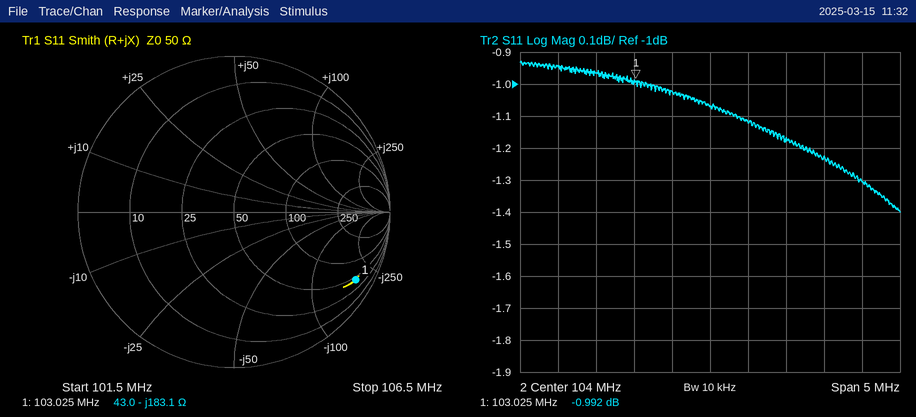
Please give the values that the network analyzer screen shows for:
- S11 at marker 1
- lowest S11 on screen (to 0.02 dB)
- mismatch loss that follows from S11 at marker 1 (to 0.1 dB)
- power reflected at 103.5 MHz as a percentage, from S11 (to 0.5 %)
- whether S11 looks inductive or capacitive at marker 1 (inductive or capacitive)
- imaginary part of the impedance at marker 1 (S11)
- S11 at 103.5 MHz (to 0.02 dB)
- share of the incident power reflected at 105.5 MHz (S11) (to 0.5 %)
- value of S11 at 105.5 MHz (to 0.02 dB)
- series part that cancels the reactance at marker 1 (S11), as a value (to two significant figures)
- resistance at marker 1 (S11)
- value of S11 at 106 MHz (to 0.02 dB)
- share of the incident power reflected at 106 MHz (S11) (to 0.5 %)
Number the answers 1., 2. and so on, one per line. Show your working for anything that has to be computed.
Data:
1. -0.992 dB
2. -1.40 dB
3. −10 log10(1 − 10^(-0.992/10)) ≈ 6.9 dB
4. 10^(-1.02/10) ≈ 79.1 %, so 79.0 % to the nearest 0.5 %
5. capacitive
6. -183.1 Ω
7. -1.02 dB
8. 10^(-1.22/10) ≈ 75.5 %
9. -1.22 dB
10. L = 183.1 Ω/(2π × 103.025 MHz) ≈ 283 nH, so 280 nH to two significant figures
11. 43.0 Ω
12. -1.30 dB
13. 10^(-1.3/10) ≈ 74.1 %, so 74.0 % to the nearest 0.5 %
